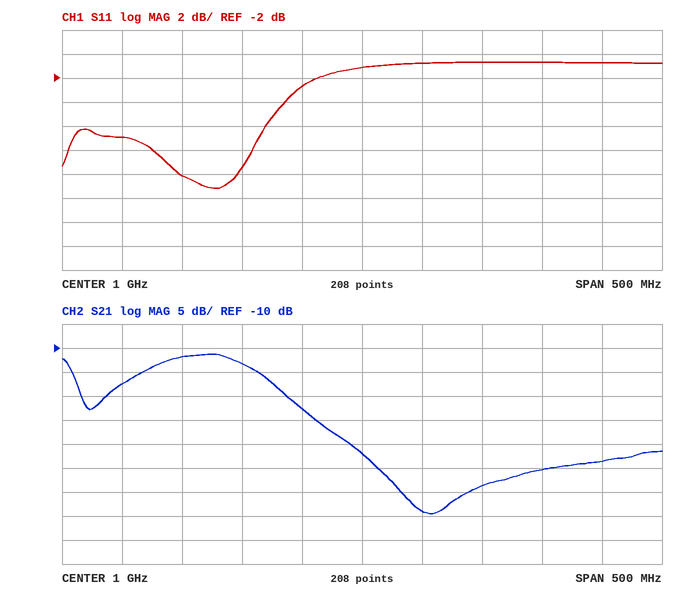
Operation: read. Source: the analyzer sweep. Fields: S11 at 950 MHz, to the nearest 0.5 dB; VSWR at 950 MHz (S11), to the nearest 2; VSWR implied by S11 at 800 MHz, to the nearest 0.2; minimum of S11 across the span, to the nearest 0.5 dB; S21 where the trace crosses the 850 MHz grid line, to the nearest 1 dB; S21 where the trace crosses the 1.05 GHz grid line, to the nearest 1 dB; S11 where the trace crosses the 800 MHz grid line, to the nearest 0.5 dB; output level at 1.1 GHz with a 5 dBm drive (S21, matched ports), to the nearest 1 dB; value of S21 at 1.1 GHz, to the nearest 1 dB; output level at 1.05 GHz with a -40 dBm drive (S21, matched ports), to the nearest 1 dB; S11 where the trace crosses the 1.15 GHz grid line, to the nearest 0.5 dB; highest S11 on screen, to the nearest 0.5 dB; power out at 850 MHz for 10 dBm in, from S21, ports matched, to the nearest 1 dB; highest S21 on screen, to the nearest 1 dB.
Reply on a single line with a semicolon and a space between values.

-2.5 dB; 6; 2.6; -11.0 dB; -12 dB; -44 dB; -7.0 dB; -34 dBm; -39 dB; -84 dBm; -0.5 dB; -0.5 dB; -2 dBm; -11 dB
